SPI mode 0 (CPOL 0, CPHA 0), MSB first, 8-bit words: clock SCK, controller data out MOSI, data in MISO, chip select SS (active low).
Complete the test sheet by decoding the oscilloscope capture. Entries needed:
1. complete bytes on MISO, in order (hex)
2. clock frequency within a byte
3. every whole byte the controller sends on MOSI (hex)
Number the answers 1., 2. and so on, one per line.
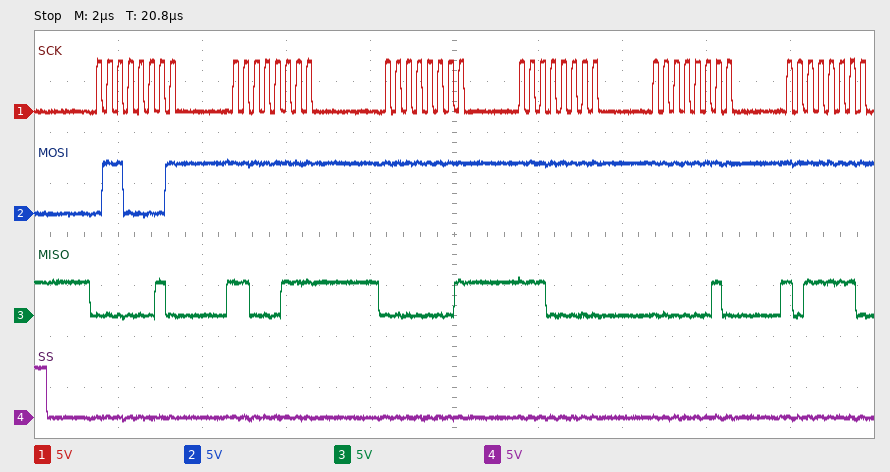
1. 02 C7 01 E0 02 BE
2. 4 MHz
3. 61 FF FF FF FF FF
